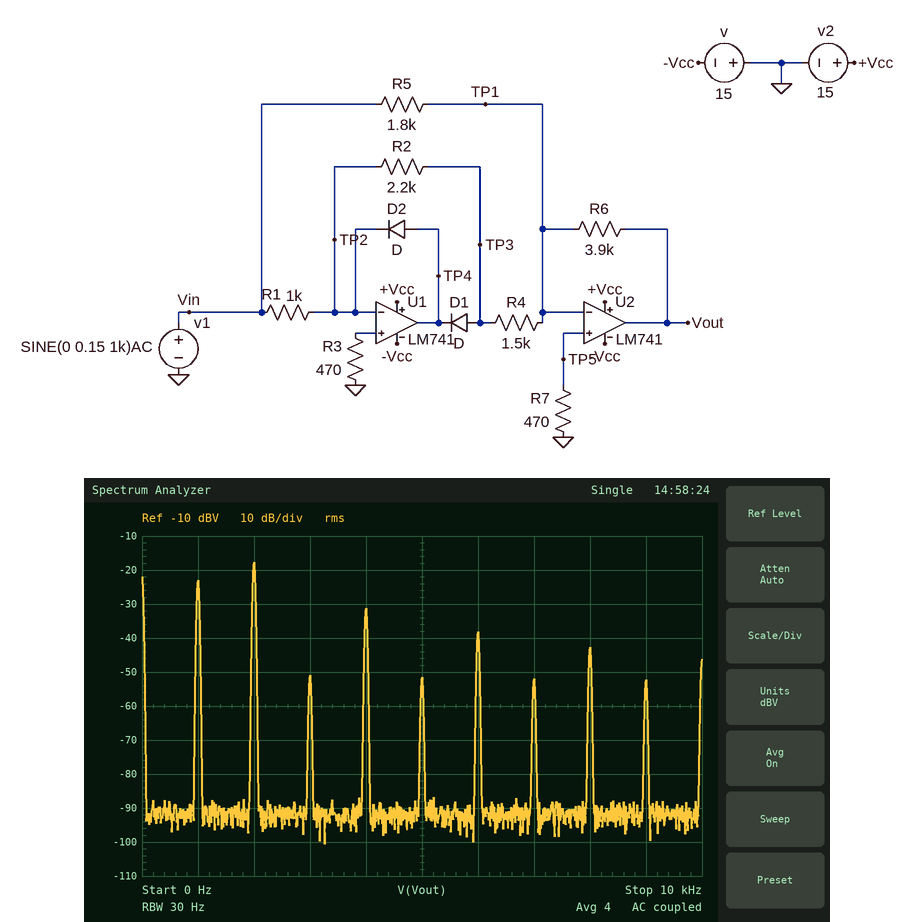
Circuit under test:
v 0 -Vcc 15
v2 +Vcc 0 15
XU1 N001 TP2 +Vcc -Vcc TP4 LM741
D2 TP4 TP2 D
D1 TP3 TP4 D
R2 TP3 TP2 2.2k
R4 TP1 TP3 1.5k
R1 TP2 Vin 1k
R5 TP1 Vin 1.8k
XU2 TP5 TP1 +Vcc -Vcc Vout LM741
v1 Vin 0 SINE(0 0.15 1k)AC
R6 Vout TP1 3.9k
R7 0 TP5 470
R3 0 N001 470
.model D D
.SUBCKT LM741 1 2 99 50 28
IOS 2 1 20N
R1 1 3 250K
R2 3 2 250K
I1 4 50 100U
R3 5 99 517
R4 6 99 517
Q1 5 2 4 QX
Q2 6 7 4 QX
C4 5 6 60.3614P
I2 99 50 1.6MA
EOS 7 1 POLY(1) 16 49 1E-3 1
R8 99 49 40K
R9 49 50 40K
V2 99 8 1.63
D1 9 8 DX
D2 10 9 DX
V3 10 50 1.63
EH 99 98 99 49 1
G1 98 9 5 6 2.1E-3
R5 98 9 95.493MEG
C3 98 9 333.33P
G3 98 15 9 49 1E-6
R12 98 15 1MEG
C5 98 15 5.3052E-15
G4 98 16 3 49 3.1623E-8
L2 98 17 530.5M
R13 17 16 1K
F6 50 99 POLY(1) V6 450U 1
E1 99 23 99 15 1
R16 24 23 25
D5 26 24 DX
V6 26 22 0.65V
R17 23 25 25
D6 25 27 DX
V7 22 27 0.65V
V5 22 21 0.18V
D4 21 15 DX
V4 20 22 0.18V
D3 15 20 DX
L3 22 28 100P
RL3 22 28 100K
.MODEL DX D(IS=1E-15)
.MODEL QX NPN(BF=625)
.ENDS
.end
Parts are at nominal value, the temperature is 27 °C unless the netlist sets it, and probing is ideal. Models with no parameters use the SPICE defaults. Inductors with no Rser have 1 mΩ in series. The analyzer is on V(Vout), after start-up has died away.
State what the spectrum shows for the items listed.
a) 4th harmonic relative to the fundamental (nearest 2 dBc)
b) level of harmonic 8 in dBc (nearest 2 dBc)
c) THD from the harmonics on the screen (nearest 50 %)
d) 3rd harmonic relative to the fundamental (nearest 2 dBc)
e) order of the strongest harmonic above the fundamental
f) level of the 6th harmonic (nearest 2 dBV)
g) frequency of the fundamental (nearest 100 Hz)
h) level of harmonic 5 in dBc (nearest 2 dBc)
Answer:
-8 dBc
-20 dBc
200 %
-28 dBc
2
-38 dBV
1.0 kHz
-28 dBc
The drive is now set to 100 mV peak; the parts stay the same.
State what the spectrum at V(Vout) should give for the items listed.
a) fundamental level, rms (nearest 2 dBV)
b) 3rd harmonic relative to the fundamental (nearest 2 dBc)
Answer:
-26 dBV
-24 dBc
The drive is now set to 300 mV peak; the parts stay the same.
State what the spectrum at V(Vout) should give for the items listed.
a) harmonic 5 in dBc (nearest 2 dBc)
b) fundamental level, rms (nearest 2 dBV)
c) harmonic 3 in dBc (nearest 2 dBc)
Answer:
-34 dBc
-16 dBV
-34 dBc
